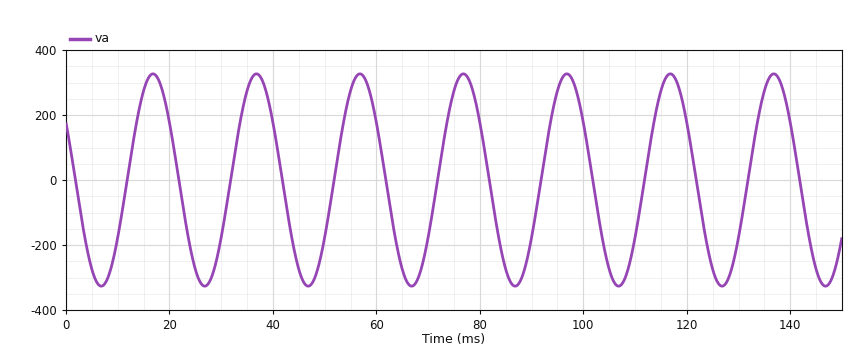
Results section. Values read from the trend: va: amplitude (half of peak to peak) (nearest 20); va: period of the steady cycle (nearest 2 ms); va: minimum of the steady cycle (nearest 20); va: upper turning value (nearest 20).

320
20 ms
-320
320
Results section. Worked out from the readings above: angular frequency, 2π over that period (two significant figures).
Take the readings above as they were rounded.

0.31 rad/ms
